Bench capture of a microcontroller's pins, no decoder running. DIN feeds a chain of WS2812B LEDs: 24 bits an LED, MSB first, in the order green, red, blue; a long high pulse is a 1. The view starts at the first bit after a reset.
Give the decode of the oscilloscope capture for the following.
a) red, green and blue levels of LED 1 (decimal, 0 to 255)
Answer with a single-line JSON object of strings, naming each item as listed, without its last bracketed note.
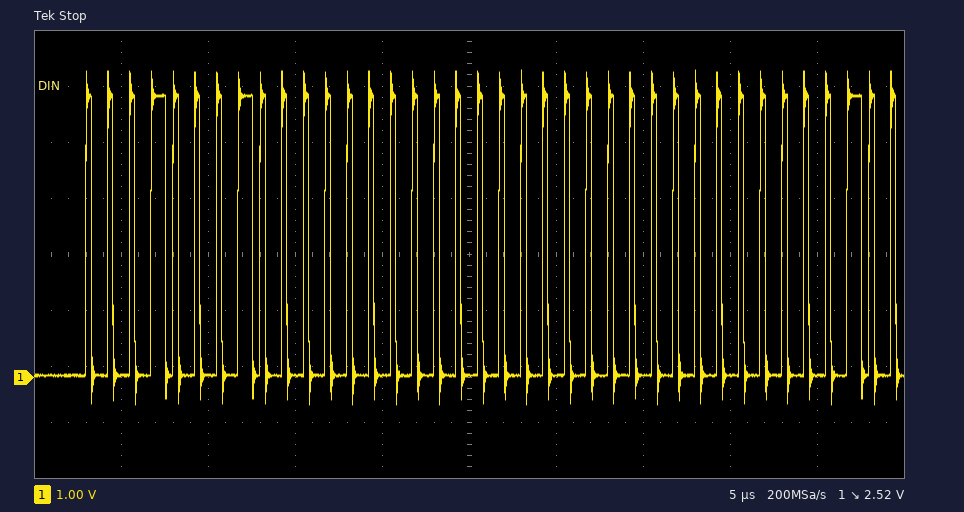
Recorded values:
{"red, green and blue levels of LED 1": "0, 17, 0"}
